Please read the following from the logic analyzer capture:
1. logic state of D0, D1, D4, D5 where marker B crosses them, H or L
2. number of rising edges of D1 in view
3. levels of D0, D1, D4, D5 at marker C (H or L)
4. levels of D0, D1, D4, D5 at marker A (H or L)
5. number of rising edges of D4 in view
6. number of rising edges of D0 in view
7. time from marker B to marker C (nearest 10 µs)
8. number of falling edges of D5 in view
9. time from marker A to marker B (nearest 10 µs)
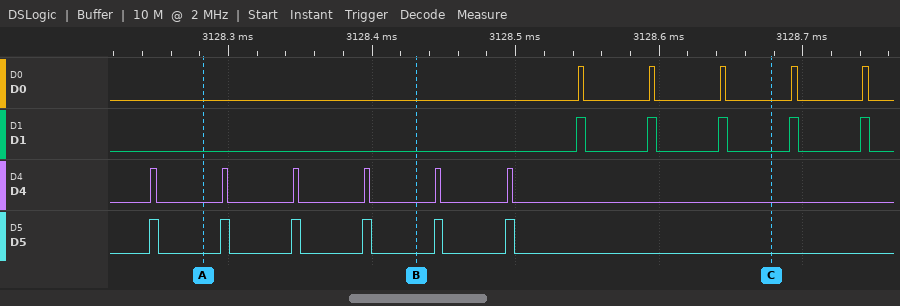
D0=L, D1=L, D4=L, D5=L
5
D0=L, D1=L, D4=L, D5=L
D0=L, D1=L, D4=L, D5=L
6
5
250 µs
6
150 µs
